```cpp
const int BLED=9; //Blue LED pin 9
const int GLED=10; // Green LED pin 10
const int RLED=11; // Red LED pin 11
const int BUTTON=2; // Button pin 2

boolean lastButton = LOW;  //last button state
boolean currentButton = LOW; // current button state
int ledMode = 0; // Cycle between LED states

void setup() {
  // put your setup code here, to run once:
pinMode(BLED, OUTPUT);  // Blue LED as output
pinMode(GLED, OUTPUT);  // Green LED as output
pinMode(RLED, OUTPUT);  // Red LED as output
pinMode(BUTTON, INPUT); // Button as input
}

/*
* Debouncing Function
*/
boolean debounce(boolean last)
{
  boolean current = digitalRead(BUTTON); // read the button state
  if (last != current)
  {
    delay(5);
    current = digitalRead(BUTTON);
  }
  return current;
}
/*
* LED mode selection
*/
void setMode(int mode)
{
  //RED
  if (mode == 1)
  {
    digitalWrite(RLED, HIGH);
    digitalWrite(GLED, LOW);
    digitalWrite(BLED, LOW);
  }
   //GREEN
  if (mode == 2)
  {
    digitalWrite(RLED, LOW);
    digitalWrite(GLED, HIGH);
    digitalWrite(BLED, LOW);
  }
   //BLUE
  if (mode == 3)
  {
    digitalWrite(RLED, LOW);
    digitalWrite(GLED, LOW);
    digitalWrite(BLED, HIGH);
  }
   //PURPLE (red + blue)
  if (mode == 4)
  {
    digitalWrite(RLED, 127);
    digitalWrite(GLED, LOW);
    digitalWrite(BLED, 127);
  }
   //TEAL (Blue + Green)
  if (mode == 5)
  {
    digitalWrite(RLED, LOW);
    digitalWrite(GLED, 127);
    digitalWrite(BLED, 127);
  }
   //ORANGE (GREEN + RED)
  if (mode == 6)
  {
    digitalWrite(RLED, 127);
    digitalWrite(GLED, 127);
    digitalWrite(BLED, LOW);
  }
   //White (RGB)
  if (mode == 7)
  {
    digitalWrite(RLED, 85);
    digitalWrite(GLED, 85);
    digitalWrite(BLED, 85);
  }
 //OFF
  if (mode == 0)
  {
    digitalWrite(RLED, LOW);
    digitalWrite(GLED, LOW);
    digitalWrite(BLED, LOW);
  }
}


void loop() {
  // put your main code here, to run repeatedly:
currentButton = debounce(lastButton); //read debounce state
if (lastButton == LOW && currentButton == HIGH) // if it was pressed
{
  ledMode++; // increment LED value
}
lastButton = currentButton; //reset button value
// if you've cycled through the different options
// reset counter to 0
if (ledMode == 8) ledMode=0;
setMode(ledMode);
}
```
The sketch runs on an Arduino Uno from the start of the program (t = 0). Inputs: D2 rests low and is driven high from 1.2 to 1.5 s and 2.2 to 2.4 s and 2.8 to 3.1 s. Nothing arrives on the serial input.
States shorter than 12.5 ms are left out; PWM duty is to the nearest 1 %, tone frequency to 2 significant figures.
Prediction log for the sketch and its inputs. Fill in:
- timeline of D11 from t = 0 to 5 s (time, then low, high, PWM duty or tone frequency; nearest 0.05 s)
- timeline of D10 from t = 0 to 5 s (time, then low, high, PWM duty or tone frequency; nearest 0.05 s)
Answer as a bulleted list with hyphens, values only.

- 0 s low; 1.2 s high; 2.2 s low
- 0 s low; 2.2 s high; 2.8 s low
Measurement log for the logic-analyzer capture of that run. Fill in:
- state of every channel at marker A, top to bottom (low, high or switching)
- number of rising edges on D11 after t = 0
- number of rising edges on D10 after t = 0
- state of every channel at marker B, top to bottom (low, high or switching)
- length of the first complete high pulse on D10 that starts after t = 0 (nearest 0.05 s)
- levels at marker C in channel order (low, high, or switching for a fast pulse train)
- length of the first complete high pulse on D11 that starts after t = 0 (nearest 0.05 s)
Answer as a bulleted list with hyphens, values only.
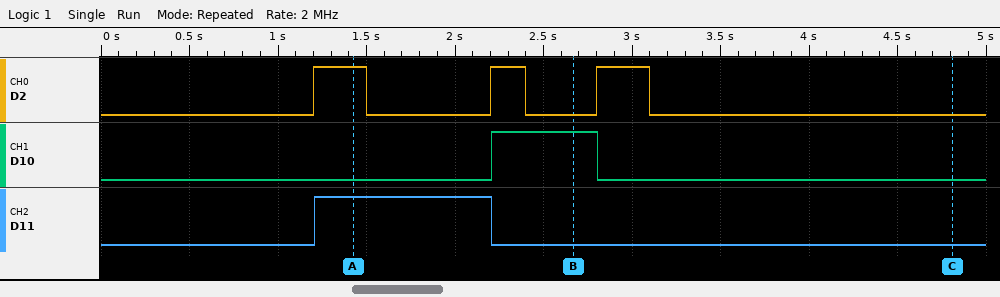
- D2 high, D10 low, D11 high
- 1
- 1
- D2 low, D10 high, D11 low
- 0.60 s
- D2 low, D10 low, D11 low
- 1.00 s
